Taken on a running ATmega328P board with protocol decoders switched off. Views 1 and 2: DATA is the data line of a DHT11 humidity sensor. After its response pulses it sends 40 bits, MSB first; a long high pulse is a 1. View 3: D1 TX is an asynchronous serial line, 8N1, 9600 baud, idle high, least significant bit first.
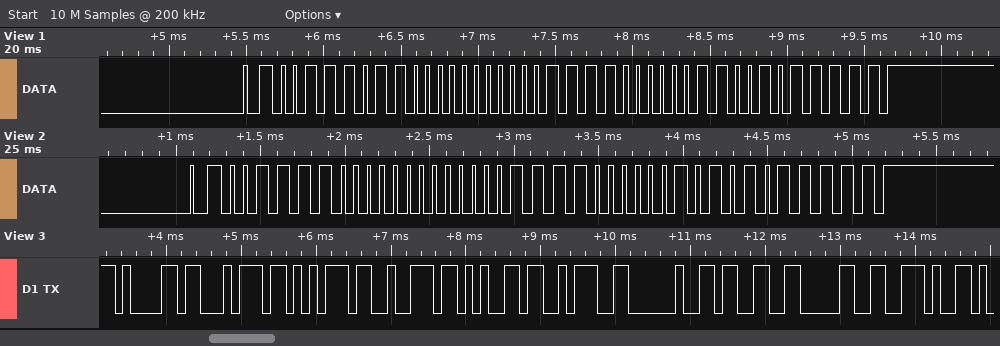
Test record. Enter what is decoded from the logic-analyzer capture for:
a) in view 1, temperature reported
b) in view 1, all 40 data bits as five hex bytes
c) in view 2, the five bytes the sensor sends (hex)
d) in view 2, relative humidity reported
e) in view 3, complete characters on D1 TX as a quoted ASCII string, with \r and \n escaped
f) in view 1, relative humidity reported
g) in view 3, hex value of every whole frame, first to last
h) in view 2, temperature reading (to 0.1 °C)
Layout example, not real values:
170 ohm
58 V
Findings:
30.6 °C
3B 00 1E 06 5F
3C 00 1E 05 5F
60 %
"ature: 30."
59 %
61 74 75 72 65 3A 20 33 30 2E
30.5 °C
